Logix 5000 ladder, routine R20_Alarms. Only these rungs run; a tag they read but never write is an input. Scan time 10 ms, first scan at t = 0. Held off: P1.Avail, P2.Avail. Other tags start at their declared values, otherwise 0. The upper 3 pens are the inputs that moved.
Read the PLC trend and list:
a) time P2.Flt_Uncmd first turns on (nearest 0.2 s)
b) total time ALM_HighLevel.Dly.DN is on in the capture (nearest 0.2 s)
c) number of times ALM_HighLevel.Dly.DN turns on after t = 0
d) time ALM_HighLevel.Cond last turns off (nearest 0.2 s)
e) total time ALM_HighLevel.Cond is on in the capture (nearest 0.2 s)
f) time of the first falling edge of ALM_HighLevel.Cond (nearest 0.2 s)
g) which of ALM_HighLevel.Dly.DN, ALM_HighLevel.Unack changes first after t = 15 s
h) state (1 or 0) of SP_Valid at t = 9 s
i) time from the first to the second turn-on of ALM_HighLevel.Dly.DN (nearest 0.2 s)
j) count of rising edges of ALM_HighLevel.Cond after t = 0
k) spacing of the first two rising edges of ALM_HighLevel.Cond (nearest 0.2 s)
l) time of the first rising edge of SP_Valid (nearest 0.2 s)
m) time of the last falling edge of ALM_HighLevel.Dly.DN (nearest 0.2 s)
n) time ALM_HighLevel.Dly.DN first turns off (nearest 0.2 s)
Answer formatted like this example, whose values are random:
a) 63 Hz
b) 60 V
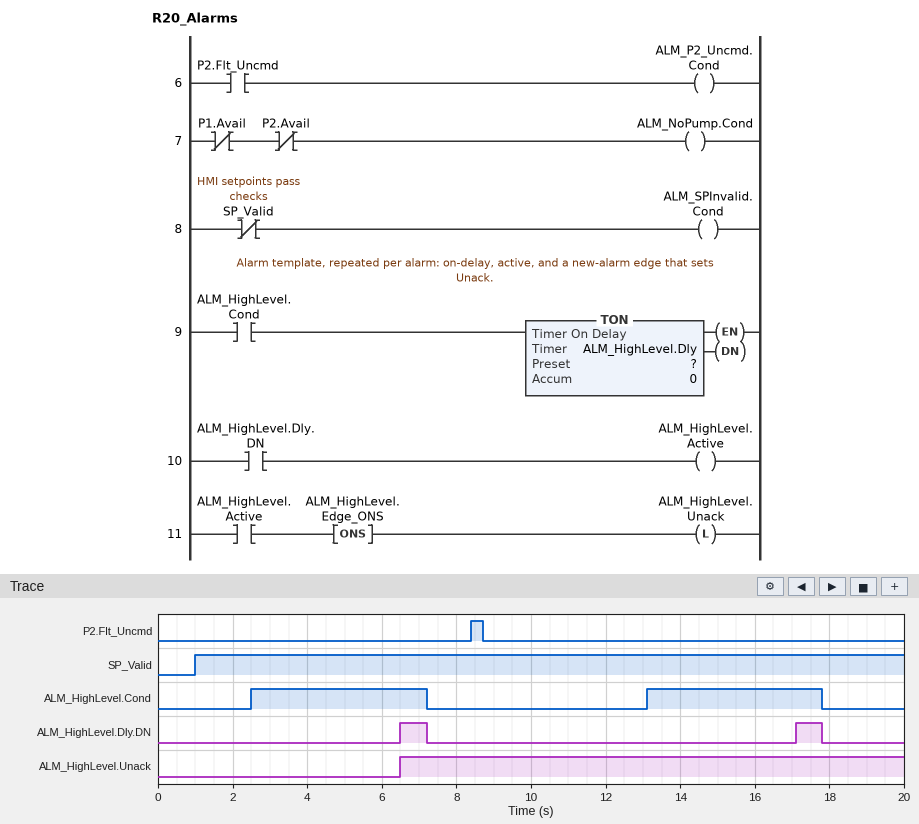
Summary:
a) 8.4 s
b) 1.4 s
c) 2
d) 17.8 s
e) 9.4 s
f) 7.2 s
g) ALM_HighLevel.Dly.DN
h) 1
i) 10.6 s
j) 2
k) 10.6 s
l) 1.0 s
m) 17.8 s
n) 7.2 s
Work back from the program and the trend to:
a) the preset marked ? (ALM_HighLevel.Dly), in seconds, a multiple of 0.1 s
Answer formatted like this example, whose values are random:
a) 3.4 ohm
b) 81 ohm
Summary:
a) 4.0 s
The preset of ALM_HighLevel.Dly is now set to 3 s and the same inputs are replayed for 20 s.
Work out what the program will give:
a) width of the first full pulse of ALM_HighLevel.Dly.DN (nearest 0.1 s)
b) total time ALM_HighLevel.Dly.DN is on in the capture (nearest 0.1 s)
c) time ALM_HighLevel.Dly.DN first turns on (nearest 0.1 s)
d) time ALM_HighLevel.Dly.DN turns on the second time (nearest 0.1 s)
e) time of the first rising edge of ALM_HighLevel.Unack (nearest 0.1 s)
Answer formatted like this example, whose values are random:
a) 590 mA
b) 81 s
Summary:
a) 1.7 s
b) 3.4 s
c) 5.5 s
d) 16.1 s
e) 5.5 s
